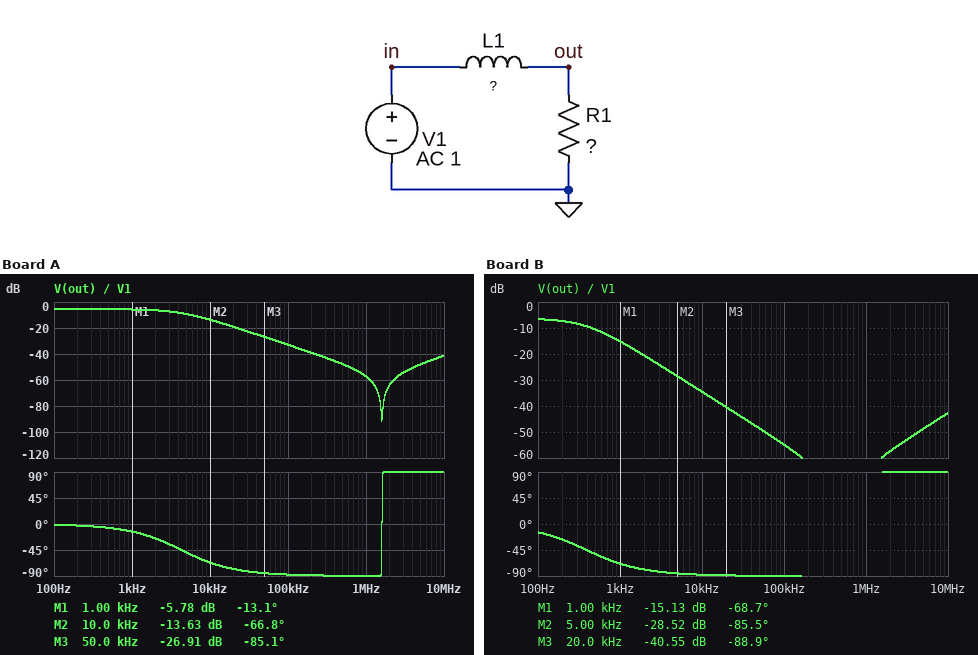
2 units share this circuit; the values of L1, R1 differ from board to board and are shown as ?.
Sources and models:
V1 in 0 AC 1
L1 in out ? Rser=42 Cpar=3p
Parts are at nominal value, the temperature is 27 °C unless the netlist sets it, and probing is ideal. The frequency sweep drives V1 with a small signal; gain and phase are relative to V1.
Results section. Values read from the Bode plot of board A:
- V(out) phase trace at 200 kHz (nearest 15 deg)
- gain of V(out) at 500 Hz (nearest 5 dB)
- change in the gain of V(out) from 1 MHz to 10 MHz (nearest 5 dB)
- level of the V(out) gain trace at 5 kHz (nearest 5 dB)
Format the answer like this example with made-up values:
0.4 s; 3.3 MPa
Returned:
-90 deg; -5 dB; 15 dB; -10 dB
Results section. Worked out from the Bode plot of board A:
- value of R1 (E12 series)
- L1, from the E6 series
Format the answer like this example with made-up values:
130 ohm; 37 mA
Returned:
47 Ω; 3.3 mH
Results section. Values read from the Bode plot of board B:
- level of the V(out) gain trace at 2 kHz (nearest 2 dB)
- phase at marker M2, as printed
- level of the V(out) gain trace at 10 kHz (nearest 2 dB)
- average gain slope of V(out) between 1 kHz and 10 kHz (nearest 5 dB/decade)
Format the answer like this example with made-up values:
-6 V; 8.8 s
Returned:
-20 dB; -85.5 deg; -34 dB; -20 dB/decade
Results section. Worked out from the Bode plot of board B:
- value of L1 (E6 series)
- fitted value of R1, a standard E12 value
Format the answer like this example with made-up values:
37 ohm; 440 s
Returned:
33 mH; 39 Ω
